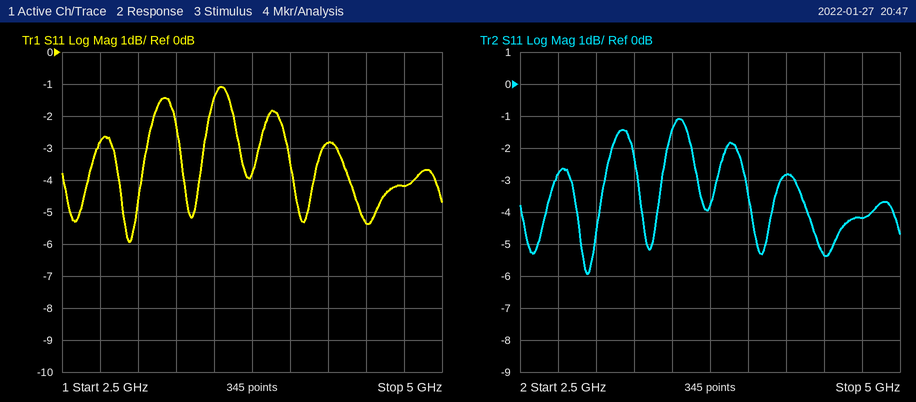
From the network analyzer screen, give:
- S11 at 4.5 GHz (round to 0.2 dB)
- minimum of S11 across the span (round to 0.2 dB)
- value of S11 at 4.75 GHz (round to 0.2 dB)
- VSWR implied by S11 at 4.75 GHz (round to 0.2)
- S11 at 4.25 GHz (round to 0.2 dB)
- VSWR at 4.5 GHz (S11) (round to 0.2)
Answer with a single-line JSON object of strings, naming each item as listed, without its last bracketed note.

{"S11 at 4.5 GHz": "-5.4 dB", "minimum of S11 across the span": "-6.0 dB", "value of S11 at 4.75 GHz": "-4.2 dB", "VSWR implied by S11 at 4.75 GHz": "4.2", "S11 at 4.25 GHz": "-2.8 dB", "VSWR at 4.5 GHz (S11)": "3.4"}
